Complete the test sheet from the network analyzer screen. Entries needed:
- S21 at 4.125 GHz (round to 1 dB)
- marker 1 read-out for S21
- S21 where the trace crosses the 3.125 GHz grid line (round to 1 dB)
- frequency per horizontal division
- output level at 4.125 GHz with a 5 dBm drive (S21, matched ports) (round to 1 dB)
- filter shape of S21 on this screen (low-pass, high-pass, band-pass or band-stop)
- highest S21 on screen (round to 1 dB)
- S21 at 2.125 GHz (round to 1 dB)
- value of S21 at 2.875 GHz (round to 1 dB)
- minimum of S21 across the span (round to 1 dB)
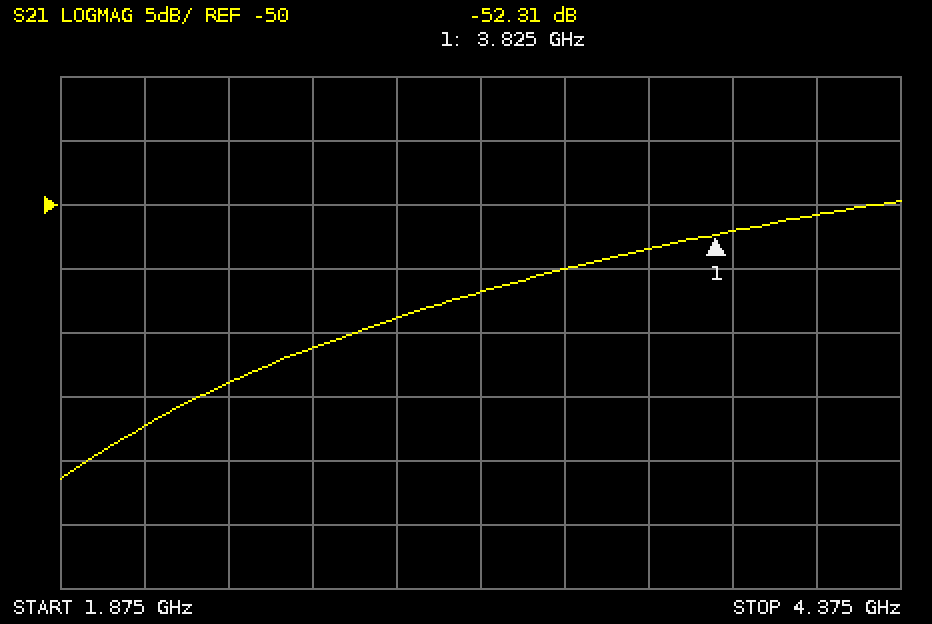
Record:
-51 dB
-52.31 dB
-57 dB
250 MHz
-46 dBm
high-pass
-50 dB
-67 dB
-59 dB
-71 dB
